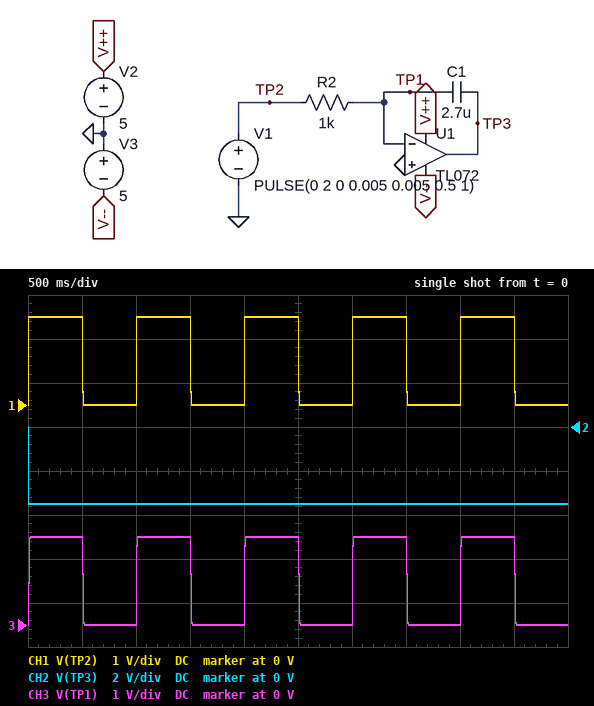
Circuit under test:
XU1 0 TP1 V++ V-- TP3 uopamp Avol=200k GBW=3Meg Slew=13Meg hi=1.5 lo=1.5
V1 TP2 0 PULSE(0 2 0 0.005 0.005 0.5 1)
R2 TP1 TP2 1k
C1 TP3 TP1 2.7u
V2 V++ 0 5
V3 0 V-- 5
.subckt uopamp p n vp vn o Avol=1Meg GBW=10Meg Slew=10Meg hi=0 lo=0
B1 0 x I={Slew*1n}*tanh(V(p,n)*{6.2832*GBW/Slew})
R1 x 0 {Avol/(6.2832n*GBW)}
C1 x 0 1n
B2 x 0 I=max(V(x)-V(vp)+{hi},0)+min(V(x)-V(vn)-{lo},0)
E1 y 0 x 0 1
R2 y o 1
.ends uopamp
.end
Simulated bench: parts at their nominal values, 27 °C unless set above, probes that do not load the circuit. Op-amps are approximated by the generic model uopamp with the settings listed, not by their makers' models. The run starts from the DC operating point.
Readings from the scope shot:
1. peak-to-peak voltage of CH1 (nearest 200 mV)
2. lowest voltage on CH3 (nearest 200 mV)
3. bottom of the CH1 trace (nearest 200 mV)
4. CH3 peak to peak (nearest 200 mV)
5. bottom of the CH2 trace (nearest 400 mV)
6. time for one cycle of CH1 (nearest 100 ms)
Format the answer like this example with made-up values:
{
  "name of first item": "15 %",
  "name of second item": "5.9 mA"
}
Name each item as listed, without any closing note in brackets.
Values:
{
  "peak-to-peak voltage of CH1": "2.0 V",
  "lowest voltage on CH3": "0 V",
  "bottom of the CH1 trace": "0 V",
  "CH3 peak to peak": "2.0 V",
  "bottom of the CH2 trace": "-3.6 V",
  "time for one cycle of CH1": "1.0 s"
}
